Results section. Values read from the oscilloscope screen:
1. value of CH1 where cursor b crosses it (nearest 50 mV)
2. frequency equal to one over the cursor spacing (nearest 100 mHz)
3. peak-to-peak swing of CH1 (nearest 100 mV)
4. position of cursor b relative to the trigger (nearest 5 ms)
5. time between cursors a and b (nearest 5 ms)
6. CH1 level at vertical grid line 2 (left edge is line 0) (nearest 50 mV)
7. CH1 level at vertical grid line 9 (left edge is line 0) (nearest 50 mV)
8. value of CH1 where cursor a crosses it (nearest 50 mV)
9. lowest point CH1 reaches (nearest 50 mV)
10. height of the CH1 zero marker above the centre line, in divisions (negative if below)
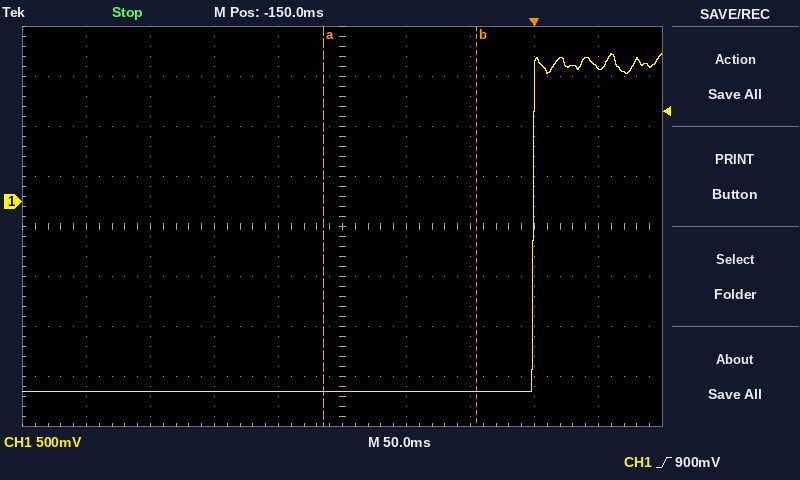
-1.90 V
8.3 Hz
3.40 V
-45 ms
120 ms
-1.90 V
1.35 V
-1.90 V
-1.90 V
+0.5 div
